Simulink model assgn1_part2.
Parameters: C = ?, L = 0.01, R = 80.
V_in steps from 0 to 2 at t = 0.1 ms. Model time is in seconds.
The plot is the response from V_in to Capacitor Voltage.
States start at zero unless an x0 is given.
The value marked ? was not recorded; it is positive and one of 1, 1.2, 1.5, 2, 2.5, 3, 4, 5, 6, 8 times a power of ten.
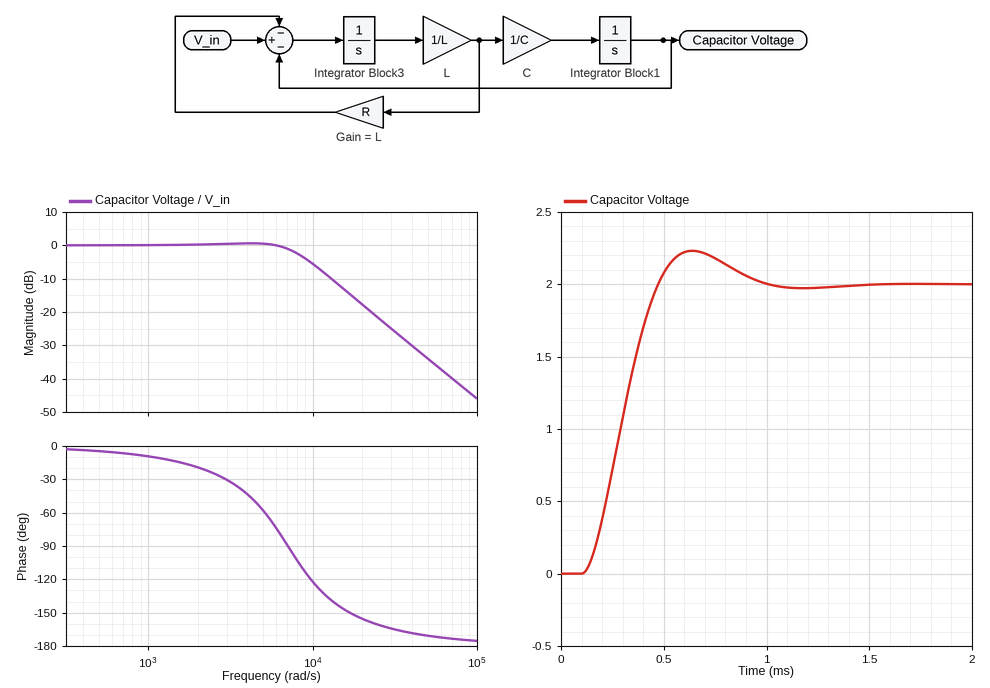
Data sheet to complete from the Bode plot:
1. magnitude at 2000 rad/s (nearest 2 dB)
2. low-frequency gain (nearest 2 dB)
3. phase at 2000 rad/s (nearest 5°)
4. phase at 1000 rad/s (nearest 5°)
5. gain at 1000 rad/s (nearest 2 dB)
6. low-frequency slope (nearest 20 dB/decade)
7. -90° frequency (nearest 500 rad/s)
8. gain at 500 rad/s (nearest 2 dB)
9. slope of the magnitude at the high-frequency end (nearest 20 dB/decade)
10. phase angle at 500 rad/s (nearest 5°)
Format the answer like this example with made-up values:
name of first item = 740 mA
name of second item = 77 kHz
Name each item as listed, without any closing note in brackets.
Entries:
magnitude at 2000 rad/s = 0 dB
low-frequency gain = 0 dB
phase at 2000 rad/s = -20°
phase at 1000 rad/s = -10°
gain at 1000 rad/s = 0 dB
low-frequency slope = 0 dB/decade
-90° frequency = 7000 rad/s
gain at 500 rad/s = 0 dB
slope of the magnitude at the high-frequency end = -40 dB/decade
phase angle at 500 rad/s = -5°
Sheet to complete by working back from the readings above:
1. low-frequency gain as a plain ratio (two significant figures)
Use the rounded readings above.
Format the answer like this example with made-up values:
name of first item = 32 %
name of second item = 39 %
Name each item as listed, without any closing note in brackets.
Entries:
low-frequency gain as a plain ratio = 1.0
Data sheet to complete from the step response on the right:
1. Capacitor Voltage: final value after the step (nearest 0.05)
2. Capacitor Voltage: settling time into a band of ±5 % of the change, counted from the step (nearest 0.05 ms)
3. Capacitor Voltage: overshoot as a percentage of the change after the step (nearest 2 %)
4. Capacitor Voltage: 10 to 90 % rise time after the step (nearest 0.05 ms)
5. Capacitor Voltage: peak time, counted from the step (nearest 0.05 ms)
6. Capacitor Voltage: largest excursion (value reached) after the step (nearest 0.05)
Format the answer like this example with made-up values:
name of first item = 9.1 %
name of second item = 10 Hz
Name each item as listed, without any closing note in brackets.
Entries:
Capacitor Voltage: final value after the step = 2.00
Capacitor Voltage: settling time into a band of ±5 % of the change, counted from the step = 0.75 ms
Capacitor Voltage: overshoot as a percentage of the change after the step = 12 %
Capacitor Voltage: 10 to 90 % rise time after the step = 0.25 ms
Capacitor Voltage: peak time, counted from the step = 0.55 ms
Capacitor Voltage: largest excursion (value reached) after the step = 2.25
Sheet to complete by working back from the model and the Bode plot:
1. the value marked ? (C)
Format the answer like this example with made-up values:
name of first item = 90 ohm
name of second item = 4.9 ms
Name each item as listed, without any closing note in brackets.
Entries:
the value marked ? = 2e-06
